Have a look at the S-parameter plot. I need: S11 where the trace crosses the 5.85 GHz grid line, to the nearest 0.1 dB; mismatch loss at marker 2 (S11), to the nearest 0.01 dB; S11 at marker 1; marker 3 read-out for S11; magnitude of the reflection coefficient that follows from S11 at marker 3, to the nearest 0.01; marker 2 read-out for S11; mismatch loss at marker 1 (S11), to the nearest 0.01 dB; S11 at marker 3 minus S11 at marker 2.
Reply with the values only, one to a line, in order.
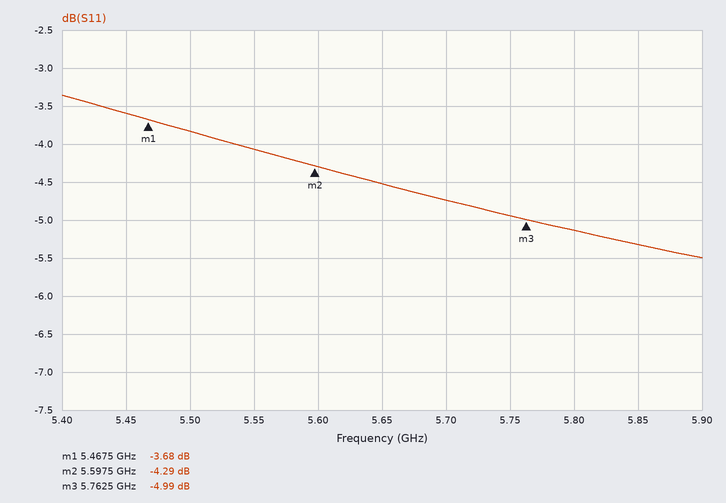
-5.3 dB
2.02 dB
-3.68 dB
-4.99 dB
0.56
-4.29 dB
2.43 dB
-0.70 dB
